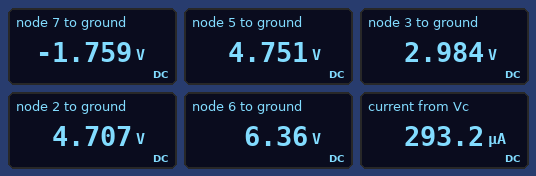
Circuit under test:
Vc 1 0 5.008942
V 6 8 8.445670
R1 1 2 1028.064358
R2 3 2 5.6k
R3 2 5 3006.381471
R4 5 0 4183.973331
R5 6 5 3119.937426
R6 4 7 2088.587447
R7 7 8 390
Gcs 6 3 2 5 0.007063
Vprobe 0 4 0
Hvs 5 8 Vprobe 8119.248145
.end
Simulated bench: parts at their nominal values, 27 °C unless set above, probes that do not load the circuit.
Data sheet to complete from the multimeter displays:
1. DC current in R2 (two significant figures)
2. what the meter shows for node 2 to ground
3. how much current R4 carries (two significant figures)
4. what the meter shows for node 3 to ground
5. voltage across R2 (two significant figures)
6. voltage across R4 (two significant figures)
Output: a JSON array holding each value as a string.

["310 µA", "4.707 V", "1.1 mA", "2.984 V", "1.7 V", "4.8 V"]
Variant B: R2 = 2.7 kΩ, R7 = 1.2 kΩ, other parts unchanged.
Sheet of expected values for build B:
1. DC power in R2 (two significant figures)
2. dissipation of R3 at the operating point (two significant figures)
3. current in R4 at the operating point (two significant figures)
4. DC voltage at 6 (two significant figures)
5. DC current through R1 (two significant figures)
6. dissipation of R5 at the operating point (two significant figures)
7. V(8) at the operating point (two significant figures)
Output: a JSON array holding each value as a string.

["72 µW", "180 nW", "1.2 mA", "5.1 V", "160 µA", "21 µW", "-3.3 V"]
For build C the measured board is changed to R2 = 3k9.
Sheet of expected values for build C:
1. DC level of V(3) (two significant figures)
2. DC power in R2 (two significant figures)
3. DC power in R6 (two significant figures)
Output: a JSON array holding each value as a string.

["3.5 V", "370 µW", "1.5 mW"]
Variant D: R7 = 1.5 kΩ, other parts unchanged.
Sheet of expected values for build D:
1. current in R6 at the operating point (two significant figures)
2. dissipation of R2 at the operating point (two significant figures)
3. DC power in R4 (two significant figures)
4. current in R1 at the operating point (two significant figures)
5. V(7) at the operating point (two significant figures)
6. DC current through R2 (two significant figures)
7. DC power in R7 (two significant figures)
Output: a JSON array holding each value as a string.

["1.1 mA", "50 µW", "5.8 mW", "90 µA", "-2.3 V", "95 µA", "1.8 mW"]
